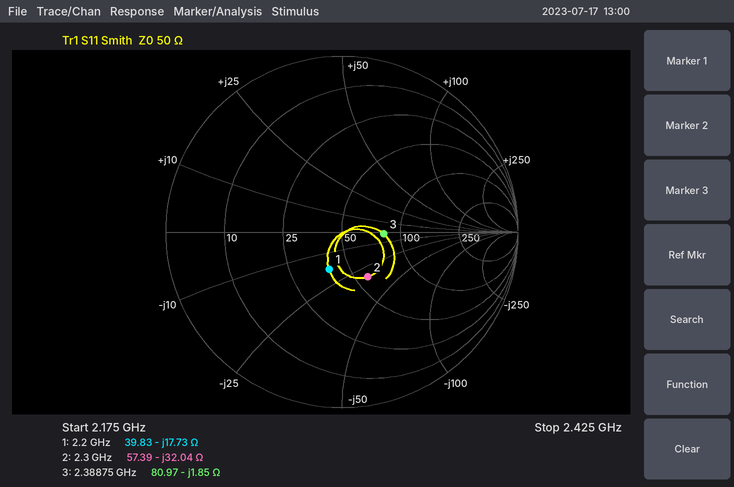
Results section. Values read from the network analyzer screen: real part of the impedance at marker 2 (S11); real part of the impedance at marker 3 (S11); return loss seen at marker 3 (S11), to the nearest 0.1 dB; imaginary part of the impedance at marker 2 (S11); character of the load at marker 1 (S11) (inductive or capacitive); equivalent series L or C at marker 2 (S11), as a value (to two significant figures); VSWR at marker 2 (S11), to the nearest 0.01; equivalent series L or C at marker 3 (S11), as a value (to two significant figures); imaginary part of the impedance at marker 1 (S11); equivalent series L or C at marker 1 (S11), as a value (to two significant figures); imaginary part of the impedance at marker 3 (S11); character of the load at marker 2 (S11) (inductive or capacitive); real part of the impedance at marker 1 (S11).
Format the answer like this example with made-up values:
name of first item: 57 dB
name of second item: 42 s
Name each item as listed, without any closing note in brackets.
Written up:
real part of the impedance at marker 2: 57.39 Ω
real part of the impedance at marker 3: 80.97 Ω
return loss seen at marker 3 (S11), to the nearest 0.1 dB: 12.5 dB
imaginary part of the impedance at marker 2: -32.04 Ω
character of the load at marker 1 (S11): capacitive
equivalent series L or C at marker 2 (S11), as a value: 2.2 pF
VSWR at marker 2 (S11), to the nearest 0.01: 1.83
equivalent series L or C at marker 3 (S11), as a value: 36 pF
imaginary part of the impedance at marker 1: -17.73 Ω
equivalent series L or C at marker 1 (S11), as a value: 4.1 pF
imaginary part of the impedance at marker 3: -1.85 Ω
character of the load at marker 2 (S11): capacitive
real part of the impedance at marker 1: 39.83 Ω
